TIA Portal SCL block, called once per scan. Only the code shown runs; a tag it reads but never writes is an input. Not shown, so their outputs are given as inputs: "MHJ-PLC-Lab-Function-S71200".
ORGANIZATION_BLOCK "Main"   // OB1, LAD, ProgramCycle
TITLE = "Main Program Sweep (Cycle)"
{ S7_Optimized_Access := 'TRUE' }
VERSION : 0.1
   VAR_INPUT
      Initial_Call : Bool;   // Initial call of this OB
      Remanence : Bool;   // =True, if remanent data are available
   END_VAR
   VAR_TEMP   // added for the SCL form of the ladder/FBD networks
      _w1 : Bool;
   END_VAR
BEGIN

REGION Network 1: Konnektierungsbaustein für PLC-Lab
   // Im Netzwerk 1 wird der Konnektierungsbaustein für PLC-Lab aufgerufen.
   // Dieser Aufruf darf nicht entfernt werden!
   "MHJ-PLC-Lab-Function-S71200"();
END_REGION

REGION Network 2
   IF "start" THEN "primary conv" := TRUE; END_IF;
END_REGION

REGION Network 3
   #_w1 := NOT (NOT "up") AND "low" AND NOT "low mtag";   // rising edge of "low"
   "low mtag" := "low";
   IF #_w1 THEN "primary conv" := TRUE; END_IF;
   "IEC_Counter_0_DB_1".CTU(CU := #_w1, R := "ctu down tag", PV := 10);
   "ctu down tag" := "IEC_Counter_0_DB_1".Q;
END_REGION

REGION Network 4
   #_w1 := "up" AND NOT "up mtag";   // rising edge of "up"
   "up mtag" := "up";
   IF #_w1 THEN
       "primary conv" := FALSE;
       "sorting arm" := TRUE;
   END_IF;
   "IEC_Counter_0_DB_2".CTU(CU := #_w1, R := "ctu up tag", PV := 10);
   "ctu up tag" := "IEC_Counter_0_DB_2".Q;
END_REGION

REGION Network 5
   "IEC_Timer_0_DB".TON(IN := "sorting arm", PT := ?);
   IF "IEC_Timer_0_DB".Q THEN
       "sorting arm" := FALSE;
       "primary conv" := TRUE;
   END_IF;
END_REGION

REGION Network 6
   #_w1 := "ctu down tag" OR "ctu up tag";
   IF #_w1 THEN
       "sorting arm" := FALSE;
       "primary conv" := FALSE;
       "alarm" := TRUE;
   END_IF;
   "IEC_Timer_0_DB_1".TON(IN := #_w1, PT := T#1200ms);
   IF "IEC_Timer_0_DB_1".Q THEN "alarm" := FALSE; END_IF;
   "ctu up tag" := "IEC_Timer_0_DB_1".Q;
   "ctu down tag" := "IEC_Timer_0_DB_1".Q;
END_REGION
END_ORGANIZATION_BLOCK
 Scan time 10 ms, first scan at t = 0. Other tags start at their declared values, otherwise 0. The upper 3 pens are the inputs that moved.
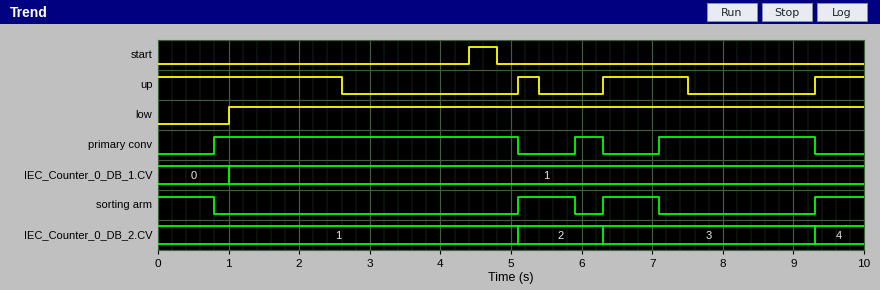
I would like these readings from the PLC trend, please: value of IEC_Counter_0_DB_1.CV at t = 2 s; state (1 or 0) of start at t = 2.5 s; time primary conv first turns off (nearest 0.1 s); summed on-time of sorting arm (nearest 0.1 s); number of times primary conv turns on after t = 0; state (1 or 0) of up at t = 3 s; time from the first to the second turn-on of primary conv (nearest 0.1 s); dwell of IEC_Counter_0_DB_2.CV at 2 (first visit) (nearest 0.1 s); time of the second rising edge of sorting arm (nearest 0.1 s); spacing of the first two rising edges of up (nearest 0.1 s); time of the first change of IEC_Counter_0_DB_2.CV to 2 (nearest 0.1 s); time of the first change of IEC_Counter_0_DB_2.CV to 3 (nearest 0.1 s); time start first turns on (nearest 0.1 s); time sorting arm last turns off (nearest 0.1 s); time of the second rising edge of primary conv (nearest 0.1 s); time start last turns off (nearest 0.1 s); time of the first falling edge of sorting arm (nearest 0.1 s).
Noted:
1
0
5.1 s
3.1 s
3
0
5.1 s
1.2 s
6.3 s
1.2 s
5.1 s
6.3 s
4.4 s
7.1 s
5.9 s
4.8 s
0.8 s
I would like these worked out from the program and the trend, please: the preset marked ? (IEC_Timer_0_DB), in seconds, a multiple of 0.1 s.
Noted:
0.8 s
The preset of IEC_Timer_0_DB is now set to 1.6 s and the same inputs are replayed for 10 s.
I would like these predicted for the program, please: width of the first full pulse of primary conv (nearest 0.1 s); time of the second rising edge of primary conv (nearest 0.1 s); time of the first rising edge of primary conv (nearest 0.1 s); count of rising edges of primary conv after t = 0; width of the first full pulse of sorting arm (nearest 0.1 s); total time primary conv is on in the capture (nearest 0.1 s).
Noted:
4.1 s
6.7 s
1.0 s
2
1.6 s
6.7 s
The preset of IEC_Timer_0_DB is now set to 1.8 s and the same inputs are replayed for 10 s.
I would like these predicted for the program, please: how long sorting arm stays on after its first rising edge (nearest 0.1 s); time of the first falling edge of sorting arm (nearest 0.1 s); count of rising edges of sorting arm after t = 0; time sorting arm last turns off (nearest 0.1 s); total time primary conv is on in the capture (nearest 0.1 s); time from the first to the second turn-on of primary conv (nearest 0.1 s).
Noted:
1.8 s
1.8 s
2
6.9 s
6.5 s
5.9 s
